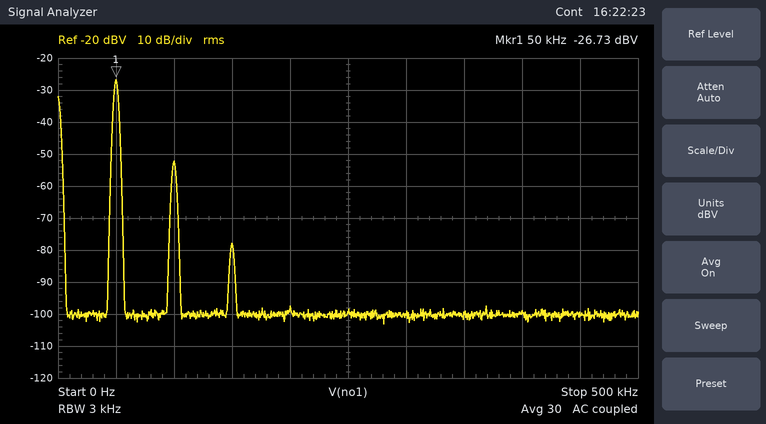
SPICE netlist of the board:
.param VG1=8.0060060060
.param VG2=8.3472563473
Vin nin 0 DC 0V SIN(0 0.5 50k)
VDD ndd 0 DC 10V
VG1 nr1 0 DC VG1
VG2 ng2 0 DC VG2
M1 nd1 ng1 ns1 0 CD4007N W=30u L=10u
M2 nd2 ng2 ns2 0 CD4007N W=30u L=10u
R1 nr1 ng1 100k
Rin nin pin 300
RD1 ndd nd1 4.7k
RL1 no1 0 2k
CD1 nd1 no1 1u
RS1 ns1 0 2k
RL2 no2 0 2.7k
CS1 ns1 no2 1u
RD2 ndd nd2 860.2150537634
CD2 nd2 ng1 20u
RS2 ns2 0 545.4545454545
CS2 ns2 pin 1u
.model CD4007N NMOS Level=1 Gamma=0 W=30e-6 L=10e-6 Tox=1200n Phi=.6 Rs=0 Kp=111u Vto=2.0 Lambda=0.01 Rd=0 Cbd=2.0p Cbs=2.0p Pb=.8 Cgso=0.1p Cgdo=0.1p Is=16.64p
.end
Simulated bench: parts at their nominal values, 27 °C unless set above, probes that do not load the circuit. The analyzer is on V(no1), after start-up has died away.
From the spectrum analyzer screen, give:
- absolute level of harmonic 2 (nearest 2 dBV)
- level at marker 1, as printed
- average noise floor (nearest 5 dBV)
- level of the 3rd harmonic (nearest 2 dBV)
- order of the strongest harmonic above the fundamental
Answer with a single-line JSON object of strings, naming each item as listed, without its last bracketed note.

{"absolute level of harmonic 2": "-52 dBV", "level at marker 1, as printed": "-26.73 dBV", "average noise floor": "-100 dBV", "level of the 3rd harmonic": "-78 dBV", "order of the strongest harmonic above the fundamental": "2"}
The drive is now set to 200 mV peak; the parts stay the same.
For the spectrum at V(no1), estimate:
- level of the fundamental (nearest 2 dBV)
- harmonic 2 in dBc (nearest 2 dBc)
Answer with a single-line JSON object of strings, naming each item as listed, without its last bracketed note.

{"level of the fundamental": "-34 dBV", "harmonic 2 in dBc": "-34 dBc"}
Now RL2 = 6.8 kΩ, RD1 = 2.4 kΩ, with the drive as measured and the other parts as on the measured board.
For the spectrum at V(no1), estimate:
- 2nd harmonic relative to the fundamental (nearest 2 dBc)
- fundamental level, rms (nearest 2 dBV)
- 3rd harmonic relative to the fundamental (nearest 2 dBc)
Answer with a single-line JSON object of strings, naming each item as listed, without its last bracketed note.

{"2nd harmonic relative to the fundamental": "-42 dBc", "fundamental level, rms": "-20 dBV", "3rd harmonic relative to the fundamental": "-58 dBc"}
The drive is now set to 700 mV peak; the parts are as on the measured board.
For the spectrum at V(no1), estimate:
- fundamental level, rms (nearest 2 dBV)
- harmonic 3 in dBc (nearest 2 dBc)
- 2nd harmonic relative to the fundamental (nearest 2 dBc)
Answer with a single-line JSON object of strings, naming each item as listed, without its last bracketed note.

{"fundamental level, rms": "-24 dBV", "harmonic 3 in dBc": "-46 dBc", "2nd harmonic relative to the fundamental": "-22 dBc"}
